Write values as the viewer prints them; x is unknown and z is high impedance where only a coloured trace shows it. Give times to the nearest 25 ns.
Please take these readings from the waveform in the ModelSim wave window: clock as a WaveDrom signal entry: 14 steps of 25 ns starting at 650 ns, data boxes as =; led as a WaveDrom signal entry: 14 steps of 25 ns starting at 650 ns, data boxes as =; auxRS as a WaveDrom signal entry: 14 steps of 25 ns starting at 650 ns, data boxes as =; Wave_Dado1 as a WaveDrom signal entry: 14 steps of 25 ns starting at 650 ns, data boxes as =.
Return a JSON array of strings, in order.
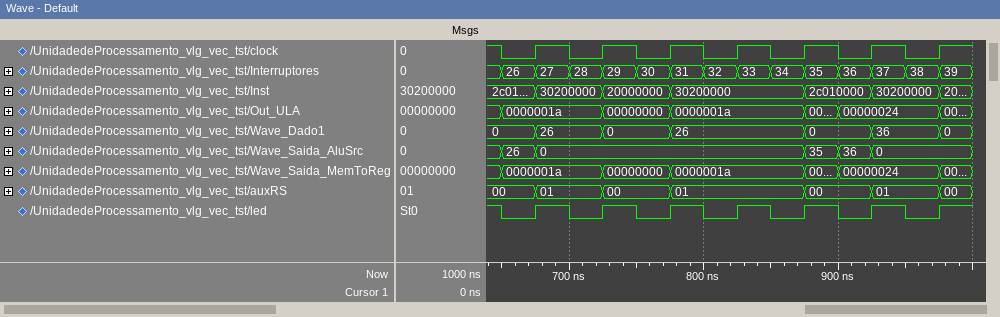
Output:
["{name: 'clock', wave: '01010101010101'}", "{name: 'led', wave: '01010101010101'}", "{name: 'auxRS', wave: '==.=.=...=.=.=', data: '00 01 00 01 00 01 00'}", "{name: 'Wave_Dado1', wave: '==.=.=...=.=.=', data: '0 26 0 26 0 36 0'}"]
